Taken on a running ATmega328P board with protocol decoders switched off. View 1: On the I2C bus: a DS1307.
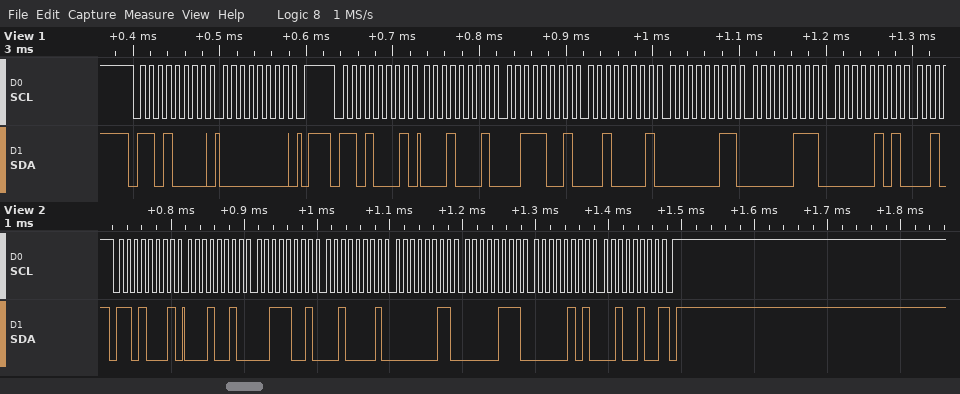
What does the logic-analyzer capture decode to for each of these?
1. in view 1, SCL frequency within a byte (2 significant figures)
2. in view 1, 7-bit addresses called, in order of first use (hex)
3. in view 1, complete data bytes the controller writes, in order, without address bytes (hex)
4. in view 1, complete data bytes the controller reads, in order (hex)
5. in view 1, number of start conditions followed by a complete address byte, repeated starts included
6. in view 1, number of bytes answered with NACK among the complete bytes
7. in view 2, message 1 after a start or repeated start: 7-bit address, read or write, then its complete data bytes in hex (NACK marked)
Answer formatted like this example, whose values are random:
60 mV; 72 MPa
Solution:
100 kHz; 0x68; 00; 11 39 21 03 07 05; 2; 0; 0x68 read: 12 39 21 03 07 05 24 NACK
